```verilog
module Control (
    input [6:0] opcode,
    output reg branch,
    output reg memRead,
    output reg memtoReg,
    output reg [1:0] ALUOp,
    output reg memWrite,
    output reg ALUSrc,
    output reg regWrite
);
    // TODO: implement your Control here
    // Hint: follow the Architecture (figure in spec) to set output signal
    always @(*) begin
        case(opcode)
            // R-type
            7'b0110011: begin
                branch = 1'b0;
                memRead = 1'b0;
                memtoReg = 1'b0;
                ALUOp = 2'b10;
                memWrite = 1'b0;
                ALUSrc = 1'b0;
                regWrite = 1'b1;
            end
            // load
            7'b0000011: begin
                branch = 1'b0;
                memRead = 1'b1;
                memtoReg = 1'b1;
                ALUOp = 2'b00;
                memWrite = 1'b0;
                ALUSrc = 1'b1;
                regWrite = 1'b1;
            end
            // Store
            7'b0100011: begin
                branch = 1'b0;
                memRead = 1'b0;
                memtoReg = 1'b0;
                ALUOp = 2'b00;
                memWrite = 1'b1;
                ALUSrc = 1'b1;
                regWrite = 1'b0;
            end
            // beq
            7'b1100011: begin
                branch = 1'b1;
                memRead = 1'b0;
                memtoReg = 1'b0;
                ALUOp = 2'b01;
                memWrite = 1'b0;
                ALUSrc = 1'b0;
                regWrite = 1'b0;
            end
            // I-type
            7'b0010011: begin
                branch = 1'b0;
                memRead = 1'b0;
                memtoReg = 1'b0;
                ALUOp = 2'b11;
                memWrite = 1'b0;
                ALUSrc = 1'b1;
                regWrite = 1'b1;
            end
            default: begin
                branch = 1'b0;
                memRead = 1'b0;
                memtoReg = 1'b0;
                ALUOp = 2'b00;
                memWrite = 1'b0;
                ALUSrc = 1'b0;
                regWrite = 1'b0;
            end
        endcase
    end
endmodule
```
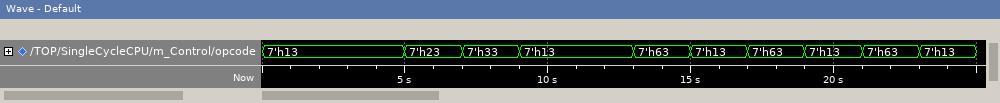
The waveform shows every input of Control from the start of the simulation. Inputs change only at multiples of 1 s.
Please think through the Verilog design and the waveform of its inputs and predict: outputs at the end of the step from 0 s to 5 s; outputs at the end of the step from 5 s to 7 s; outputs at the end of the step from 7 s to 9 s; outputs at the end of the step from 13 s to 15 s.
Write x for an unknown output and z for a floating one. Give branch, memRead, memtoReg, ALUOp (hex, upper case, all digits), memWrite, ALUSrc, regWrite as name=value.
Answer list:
branch=0, memRead=0, memtoReg=0, ALUOp=3, memWrite=0, ALUSrc=1, regWrite=1
branch=0, memRead=0, memtoReg=0, ALUOp=0, memWrite=1, ALUSrc=1, regWrite=0
branch=0, memRead=0, memtoReg=0, ALUOp=2, memWrite=0, ALUSrc=0, regWrite=1
branch=1, memRead=0, memtoReg=0, ALUOp=1, memWrite=0, ALUSrc=0, regWrite=0
